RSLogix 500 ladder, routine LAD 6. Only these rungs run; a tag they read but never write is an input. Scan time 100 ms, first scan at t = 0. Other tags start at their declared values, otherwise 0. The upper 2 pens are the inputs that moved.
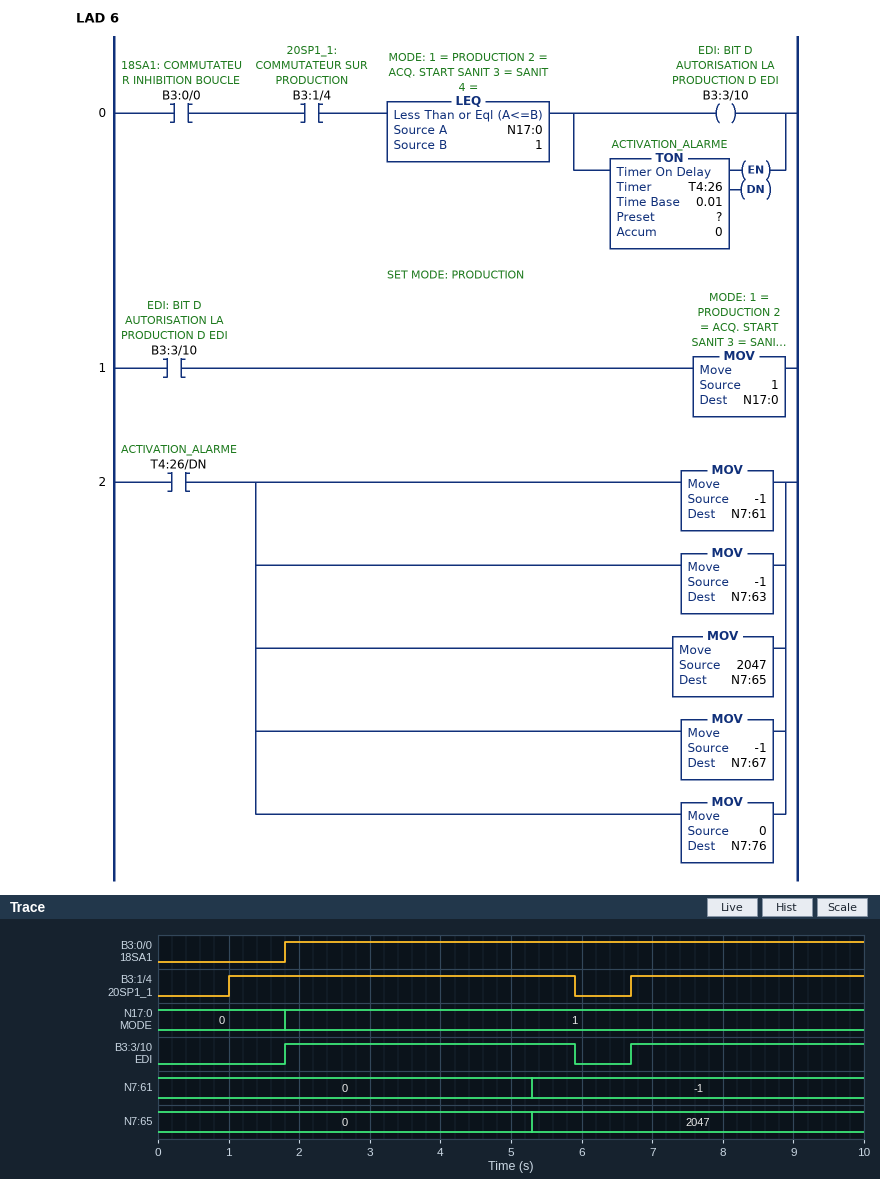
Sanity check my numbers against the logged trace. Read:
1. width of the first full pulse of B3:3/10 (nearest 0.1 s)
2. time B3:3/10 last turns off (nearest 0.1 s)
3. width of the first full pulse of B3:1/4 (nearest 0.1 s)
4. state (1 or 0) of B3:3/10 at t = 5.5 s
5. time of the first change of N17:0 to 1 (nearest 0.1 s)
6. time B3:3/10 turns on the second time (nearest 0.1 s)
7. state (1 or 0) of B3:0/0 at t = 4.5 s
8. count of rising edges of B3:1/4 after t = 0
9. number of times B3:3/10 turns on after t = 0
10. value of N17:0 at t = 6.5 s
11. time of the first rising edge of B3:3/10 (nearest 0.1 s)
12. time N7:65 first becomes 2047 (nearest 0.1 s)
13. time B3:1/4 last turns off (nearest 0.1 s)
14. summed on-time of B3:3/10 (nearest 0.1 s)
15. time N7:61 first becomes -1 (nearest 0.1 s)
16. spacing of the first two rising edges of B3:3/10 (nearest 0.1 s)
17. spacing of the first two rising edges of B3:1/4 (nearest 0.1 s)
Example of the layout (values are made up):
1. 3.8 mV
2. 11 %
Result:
1. 4.1 s
2. 5.9 s
3. 4.9 s
4. 1
5. 1.8 s
6. 6.7 s
7. 1
8. 2
9. 2
10. 1
11. 1.8 s
12. 5.3 s
13. 5.9 s
14. 7.4 s
15. 5.3 s
16. 4.9 s
17. 5.7 s
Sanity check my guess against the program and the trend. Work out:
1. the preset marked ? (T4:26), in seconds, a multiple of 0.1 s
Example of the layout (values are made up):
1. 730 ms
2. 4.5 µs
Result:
1. 3.5 s
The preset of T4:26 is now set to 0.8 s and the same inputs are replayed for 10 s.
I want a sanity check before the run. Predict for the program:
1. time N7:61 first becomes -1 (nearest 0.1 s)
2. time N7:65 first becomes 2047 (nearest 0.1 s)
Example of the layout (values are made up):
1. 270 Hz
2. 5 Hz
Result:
1. 2.6 s
2. 2.6 s
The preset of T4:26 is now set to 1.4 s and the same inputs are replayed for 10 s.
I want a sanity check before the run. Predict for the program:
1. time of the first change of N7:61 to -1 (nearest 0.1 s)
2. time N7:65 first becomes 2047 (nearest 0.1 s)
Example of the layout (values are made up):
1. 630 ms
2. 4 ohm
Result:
1. 3.2 s
2. 3.2 s
